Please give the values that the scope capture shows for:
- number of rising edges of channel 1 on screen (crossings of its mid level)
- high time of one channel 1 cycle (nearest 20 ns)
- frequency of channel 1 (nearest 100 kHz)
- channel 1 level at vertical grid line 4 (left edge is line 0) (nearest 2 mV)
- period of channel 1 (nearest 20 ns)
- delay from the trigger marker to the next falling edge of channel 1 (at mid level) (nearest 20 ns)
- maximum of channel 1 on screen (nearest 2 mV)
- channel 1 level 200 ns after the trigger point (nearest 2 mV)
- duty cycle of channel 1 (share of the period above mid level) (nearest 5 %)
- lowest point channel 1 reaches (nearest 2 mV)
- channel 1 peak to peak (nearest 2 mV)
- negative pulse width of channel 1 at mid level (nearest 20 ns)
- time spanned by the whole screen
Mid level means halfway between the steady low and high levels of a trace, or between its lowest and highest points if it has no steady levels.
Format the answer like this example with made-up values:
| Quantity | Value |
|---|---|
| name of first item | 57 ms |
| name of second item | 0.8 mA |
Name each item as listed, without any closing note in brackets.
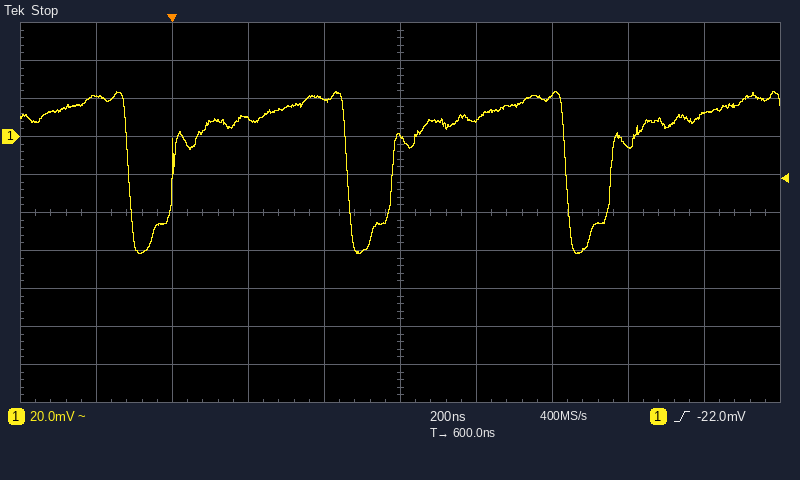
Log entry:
| Quantity | Value |
|---|---|
| number of rising edges of channel 1 on screen | 3 |
| high time of one channel 1 cycle | 460 ns |
| frequency of channel 1 | 1.7 MHz |
| channel 1 level at vertical grid line 4 (left edge is line 0) | 20 mV |
| period of channel 1 | 580 ns |
| delay from the trigger marker to the next falling edge of channel 1 (at mid level) | 460 ns |
| maximum of channel 1 on screen | 24 mV |
| channel 1 level 200 ns after the trigger point | 10 mV |
| duty cycle of channel 1 (share of the period above mid level) | 80 % |
| lowest point channel 1 reaches | -62 mV |
| channel 1 peak to peak | 86 mV |
| negative pulse width of channel 1 at mid level | 120 ns |
| time spanned by the whole screen | 2 µs |
